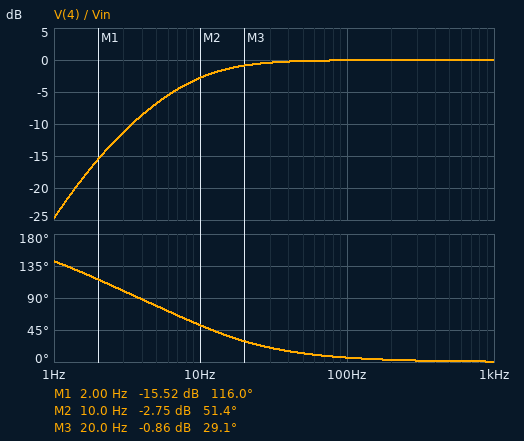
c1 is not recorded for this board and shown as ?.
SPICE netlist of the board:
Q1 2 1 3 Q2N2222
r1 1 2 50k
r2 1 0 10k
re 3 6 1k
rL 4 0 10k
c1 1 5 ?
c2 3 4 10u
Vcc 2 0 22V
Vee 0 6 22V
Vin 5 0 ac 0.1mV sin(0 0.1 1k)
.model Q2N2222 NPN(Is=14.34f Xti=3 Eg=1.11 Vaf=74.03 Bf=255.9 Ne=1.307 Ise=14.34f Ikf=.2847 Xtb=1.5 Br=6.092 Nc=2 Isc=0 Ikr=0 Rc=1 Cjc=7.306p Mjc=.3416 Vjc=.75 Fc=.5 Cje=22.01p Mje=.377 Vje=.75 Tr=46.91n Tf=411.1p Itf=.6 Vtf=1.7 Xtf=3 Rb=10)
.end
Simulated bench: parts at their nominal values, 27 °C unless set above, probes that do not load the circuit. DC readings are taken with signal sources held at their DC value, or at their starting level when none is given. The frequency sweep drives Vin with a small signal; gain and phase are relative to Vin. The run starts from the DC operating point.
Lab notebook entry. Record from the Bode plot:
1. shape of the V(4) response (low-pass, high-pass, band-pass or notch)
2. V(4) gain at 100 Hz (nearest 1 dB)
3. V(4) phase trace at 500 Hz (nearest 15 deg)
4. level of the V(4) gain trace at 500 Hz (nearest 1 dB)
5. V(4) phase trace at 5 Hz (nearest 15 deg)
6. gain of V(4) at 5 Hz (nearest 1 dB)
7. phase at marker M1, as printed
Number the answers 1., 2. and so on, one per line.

1. high-pass
2. 0 dB
3. 0 deg
4. 0 dB
5. 75 deg
6. -7 dB
7. 116.0 deg
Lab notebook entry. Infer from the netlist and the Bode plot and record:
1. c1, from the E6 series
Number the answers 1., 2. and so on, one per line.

1. 2.2 µF
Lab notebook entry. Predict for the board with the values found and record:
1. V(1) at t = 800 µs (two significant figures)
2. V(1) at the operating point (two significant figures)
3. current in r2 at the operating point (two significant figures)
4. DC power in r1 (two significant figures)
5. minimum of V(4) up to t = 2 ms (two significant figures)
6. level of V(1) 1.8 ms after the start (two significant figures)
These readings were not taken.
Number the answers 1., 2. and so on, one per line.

1. 2.7 V
2. 2.8 V
3. 280 µA
4. 7.4 mW
5. -100 mV
6. 2.7 V
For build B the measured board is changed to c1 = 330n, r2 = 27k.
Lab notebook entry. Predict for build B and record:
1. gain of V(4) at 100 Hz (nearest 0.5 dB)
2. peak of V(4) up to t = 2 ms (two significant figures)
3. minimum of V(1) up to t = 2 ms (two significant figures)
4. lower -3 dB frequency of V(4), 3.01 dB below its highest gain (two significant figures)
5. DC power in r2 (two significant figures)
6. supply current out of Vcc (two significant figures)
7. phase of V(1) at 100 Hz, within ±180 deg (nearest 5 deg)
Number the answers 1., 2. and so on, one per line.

1. -0.5 dB
2. 97 mV
3. 5.4 V
4. 31 Hz
5. 1.1 mW
6. 27 mA
7. 15 deg
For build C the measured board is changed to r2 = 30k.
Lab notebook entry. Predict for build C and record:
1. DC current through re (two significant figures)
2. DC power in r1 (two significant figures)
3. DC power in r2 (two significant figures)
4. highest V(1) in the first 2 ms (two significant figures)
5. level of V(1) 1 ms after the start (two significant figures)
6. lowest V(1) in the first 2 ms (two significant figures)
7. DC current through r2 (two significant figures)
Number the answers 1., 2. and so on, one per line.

1. 27 mA
2. 5.2 mW
3. 1.2 mW
4. 6.0 V
5. 5.9 V
6. 5.8 V
7. 200 µA
